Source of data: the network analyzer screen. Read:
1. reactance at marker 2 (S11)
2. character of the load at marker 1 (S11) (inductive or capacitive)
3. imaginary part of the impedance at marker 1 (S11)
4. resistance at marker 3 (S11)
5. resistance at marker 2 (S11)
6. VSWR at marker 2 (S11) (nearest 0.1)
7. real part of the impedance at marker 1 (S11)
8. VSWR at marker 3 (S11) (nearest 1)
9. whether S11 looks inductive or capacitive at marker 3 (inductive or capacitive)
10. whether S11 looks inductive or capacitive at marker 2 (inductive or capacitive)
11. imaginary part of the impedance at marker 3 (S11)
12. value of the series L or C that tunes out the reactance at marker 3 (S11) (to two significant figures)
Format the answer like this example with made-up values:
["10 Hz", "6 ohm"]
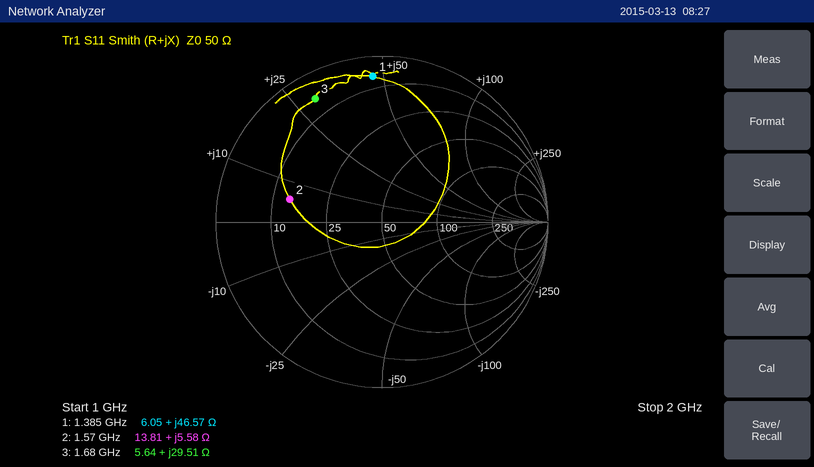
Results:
["+5.58 Ω", "inductive", "+46.57 Ω", "5.64 Ω", "13.81 Ω", "3.7", "6.05 Ω", "12", "inductive", "inductive", "+29.51 Ω", "3.2 pF"]
